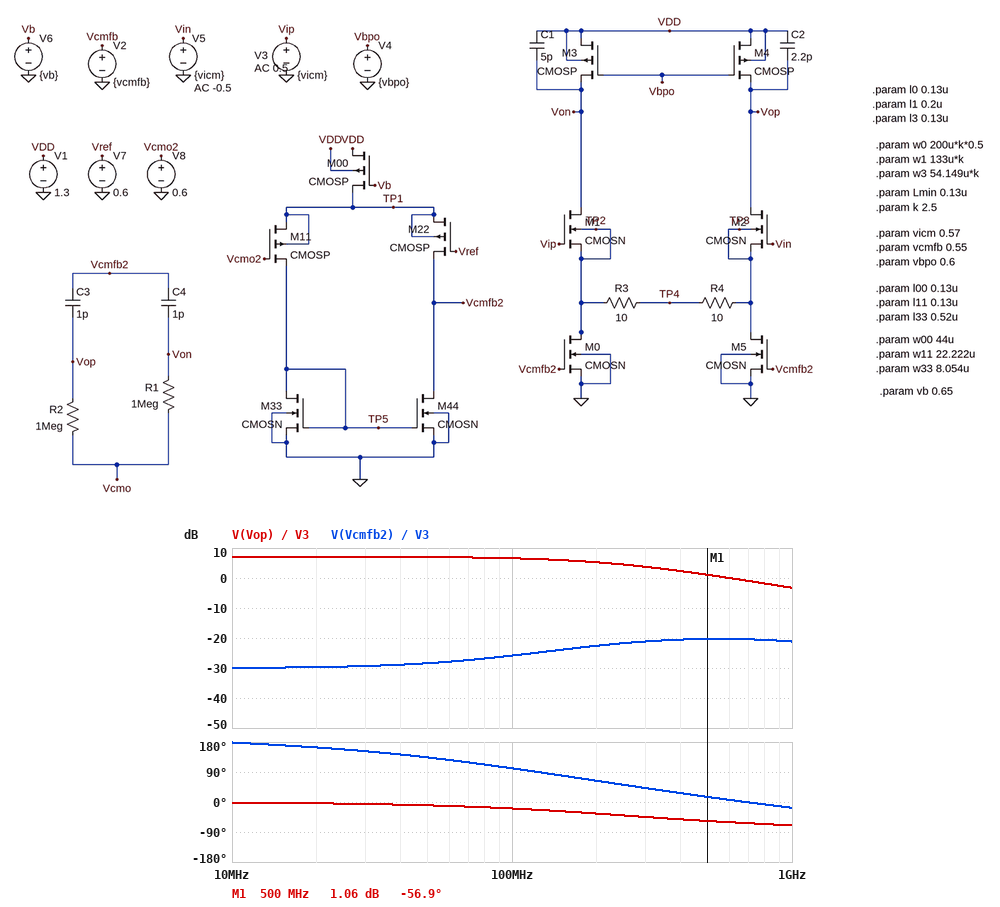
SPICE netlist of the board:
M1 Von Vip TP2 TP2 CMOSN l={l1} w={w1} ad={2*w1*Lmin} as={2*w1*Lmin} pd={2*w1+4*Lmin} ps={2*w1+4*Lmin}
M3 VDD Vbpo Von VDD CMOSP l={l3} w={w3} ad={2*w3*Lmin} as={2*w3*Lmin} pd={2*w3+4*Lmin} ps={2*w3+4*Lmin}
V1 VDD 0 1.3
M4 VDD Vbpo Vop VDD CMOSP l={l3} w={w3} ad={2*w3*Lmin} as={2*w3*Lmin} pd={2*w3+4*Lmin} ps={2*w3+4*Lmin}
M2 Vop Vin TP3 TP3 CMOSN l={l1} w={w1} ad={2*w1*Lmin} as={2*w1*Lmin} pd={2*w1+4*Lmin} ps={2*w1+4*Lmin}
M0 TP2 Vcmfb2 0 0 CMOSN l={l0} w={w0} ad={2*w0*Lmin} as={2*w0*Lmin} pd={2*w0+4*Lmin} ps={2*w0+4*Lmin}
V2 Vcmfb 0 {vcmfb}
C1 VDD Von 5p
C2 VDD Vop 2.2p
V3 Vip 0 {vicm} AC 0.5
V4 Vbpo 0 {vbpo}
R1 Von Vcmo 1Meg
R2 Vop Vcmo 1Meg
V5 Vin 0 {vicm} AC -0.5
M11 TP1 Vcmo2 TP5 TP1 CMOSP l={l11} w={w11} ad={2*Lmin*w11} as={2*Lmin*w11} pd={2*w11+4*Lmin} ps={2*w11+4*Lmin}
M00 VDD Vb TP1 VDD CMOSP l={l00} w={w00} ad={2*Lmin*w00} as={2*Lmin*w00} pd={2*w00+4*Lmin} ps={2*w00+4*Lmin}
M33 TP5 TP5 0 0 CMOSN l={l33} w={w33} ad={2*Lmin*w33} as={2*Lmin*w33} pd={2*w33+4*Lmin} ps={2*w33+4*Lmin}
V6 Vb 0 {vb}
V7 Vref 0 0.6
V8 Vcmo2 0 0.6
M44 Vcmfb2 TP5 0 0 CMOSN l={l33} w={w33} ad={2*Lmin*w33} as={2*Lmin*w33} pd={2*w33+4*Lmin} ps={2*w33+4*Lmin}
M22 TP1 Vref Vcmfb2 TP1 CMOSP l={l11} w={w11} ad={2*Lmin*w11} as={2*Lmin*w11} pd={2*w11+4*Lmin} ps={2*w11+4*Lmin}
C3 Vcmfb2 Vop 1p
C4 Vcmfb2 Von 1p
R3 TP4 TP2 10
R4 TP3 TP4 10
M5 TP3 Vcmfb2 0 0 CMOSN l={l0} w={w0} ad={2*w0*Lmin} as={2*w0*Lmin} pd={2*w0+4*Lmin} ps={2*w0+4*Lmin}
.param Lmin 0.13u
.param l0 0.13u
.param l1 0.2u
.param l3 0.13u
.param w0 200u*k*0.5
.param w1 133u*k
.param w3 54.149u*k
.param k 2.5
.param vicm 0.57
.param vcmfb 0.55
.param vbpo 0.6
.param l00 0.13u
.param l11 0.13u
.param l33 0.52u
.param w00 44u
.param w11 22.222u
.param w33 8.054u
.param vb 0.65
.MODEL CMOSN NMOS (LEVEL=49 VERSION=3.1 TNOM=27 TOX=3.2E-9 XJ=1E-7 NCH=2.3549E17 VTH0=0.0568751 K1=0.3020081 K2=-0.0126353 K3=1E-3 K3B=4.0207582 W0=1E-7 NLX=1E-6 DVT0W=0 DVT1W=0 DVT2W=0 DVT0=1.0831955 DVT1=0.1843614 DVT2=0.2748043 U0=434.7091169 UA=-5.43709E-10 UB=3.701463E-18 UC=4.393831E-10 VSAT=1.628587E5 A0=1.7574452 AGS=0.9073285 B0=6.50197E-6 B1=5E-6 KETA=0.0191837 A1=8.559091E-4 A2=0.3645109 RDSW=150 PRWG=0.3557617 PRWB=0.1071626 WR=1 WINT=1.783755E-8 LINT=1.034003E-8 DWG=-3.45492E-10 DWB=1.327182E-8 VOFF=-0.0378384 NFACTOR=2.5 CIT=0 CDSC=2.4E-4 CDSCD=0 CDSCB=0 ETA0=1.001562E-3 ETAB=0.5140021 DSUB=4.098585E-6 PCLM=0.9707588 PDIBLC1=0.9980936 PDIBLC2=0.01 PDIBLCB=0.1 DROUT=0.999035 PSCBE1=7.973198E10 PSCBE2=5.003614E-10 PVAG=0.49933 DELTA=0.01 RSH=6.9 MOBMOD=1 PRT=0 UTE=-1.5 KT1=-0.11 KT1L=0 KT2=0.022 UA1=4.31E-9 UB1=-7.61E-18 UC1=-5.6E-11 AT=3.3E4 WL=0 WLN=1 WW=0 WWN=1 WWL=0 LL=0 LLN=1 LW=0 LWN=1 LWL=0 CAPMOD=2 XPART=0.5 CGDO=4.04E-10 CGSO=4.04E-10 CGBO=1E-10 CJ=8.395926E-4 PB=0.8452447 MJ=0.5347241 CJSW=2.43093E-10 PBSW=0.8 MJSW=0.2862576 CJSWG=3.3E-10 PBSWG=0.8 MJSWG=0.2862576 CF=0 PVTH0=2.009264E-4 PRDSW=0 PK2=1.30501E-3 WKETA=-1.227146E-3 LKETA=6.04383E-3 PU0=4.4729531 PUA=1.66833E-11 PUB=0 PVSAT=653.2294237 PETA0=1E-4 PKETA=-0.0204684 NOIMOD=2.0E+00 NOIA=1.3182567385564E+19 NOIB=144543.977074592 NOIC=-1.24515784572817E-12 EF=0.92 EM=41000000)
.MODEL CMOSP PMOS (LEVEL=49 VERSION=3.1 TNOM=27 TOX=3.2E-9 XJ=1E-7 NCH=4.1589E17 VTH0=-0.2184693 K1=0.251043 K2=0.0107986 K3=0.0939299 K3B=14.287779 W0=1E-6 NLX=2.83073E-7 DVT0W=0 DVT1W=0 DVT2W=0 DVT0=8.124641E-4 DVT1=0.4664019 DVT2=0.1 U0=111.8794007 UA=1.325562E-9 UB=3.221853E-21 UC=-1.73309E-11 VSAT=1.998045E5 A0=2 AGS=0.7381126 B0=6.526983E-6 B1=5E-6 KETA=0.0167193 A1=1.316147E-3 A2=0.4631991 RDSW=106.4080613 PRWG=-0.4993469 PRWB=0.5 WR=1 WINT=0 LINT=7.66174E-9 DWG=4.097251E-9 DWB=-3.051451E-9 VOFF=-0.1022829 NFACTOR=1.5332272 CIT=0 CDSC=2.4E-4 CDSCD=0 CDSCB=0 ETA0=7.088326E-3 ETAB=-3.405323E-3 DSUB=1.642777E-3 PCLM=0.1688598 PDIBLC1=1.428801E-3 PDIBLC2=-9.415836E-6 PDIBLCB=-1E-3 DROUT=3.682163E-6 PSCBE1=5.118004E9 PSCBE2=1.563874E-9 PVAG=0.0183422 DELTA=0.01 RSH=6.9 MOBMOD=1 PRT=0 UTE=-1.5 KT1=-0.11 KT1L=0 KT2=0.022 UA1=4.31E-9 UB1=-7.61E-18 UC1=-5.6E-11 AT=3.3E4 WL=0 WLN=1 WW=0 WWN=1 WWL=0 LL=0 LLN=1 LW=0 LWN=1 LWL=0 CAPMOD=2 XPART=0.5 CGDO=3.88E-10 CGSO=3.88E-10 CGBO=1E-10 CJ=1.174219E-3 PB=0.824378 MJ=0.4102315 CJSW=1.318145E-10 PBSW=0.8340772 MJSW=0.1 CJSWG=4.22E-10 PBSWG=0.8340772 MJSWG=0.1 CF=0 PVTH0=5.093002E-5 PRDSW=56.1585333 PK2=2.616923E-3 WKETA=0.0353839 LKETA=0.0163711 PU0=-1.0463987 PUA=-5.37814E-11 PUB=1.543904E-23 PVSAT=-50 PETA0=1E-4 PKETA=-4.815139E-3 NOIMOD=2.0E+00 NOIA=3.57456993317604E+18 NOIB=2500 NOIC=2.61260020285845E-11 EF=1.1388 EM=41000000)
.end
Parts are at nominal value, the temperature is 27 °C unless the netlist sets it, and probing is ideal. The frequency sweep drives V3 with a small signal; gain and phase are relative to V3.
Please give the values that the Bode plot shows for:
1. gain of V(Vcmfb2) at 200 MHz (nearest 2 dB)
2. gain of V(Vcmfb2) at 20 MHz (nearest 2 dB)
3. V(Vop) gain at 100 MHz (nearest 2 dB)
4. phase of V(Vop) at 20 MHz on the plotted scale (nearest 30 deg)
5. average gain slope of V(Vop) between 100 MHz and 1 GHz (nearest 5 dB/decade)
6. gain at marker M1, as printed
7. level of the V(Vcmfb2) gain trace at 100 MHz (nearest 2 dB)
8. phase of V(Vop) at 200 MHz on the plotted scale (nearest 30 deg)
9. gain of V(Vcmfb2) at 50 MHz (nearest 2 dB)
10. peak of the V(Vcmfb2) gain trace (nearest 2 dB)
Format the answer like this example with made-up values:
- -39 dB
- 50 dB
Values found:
- -22 dB
- -30 dB
- 6 dB
- 0 deg
- -10 dB/decade
- 1.06 dB
- -26 dB
- -30 deg
- -28 dB
- -20 dB
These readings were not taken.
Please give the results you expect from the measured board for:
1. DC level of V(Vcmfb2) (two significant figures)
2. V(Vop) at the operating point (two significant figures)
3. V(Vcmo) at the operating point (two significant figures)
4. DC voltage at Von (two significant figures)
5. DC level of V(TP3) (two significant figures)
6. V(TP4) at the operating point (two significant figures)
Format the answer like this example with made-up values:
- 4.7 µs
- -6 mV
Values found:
- 550 mV
- 1.1 V
- 1.1 V
- 1.1 V
- 130 mV
- 130 mV
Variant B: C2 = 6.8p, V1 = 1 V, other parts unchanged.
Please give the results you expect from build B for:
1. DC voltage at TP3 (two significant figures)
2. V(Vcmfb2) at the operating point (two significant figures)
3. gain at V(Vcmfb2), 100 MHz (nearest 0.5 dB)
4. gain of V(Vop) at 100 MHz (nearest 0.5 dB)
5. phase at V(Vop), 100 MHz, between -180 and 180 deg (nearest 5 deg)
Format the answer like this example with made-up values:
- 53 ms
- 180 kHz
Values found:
- 390 mV
- 260 mV
- -38.0 dB
- -31.5 dB
- -90 deg
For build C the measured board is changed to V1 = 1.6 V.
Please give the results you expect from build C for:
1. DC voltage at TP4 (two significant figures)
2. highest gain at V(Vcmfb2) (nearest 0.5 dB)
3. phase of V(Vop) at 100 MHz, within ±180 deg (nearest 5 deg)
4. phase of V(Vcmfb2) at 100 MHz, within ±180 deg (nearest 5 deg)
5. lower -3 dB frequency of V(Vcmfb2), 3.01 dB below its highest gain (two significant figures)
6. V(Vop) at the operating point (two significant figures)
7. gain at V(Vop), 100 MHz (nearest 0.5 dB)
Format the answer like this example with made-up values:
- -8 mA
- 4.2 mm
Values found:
- 85 mV
- -16.0 dB
- -5 deg
- 170 deg
- 14 MHz
- 1.4 V
- -0.5 dB
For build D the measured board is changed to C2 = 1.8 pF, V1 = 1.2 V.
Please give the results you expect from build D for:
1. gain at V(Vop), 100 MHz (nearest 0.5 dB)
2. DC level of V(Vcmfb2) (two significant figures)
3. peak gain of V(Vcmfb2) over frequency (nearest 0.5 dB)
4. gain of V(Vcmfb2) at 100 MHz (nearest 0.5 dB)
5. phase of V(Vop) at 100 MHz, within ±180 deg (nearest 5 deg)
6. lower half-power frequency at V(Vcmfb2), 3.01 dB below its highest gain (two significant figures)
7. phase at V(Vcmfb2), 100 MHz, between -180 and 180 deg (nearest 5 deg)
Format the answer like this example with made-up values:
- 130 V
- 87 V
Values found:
- -2.5 dB
- 450 mV
- -22.5 dB
- -30.5 dB
- -15 deg
- 210 MHz
- 65 deg
